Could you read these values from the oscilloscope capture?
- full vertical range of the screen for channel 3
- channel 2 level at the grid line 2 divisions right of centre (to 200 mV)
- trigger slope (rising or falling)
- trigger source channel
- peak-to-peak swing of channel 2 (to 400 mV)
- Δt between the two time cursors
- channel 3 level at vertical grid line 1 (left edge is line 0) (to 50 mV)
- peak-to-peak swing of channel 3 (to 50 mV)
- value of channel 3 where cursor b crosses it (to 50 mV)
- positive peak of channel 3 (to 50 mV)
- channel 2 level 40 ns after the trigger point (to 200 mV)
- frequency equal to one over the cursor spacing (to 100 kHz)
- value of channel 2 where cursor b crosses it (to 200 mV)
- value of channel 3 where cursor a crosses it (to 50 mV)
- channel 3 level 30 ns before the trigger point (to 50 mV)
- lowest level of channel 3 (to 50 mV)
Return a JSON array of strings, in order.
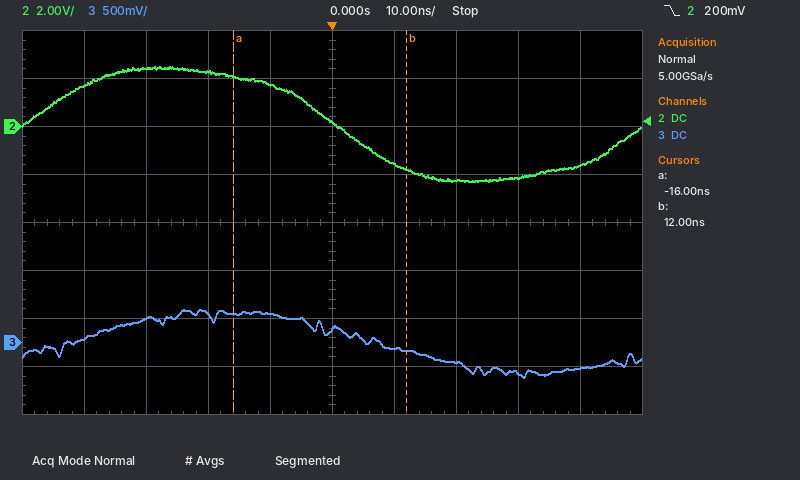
["4 V", "-2.2 V", "falling", "channel 2", "4.8 V", "28 ns", "50 mV", "700 mV", "-100 mV", "350 mV", "-1.6 V", "35.7 MHz", "-1.8 V", "300 mV", "250 mV", "-350 mV"]
